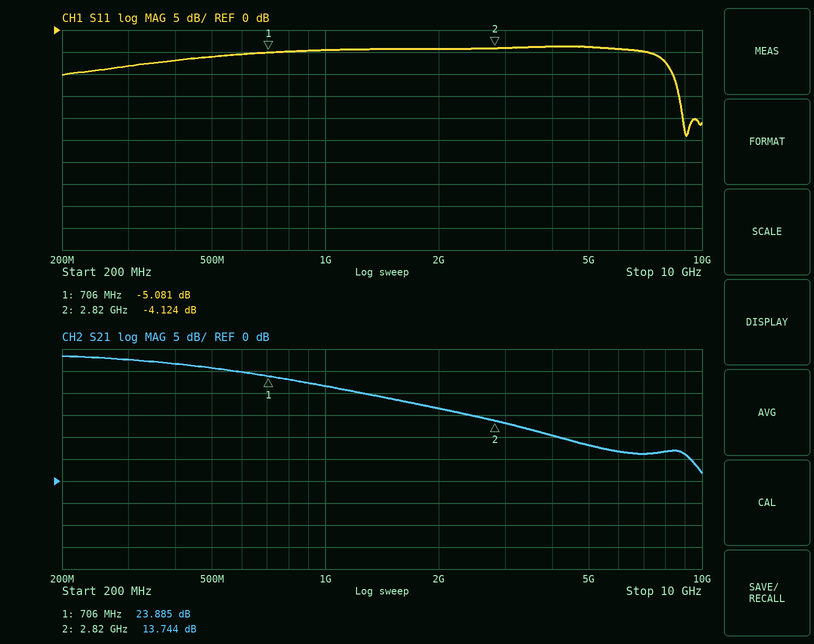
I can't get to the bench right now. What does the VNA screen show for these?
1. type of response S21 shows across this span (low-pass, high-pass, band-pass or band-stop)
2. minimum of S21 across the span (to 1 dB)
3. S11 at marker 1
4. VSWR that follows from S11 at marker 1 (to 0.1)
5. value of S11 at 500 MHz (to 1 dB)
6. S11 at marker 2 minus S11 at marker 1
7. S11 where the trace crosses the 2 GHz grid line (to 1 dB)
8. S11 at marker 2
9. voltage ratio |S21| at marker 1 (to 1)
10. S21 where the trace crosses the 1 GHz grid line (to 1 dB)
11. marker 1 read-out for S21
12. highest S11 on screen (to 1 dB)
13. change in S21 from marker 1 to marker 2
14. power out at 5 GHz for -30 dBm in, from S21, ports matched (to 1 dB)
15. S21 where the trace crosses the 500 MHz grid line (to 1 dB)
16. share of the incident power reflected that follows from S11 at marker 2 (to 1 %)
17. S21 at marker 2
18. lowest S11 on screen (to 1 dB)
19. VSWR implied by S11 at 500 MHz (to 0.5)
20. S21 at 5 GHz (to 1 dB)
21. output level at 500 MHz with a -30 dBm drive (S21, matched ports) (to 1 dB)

low-pass
2 dB
-5.081 dB
3.5
-6 dB
0.957 dB
-4 dB
-4.124 dB
16
22 dB
23.885 dB
-4 dB
-10.141 dB
-22 dBm
26 dB
39 %
13.744 dB
-24 dB
3.0
8 dB
-4 dBm
